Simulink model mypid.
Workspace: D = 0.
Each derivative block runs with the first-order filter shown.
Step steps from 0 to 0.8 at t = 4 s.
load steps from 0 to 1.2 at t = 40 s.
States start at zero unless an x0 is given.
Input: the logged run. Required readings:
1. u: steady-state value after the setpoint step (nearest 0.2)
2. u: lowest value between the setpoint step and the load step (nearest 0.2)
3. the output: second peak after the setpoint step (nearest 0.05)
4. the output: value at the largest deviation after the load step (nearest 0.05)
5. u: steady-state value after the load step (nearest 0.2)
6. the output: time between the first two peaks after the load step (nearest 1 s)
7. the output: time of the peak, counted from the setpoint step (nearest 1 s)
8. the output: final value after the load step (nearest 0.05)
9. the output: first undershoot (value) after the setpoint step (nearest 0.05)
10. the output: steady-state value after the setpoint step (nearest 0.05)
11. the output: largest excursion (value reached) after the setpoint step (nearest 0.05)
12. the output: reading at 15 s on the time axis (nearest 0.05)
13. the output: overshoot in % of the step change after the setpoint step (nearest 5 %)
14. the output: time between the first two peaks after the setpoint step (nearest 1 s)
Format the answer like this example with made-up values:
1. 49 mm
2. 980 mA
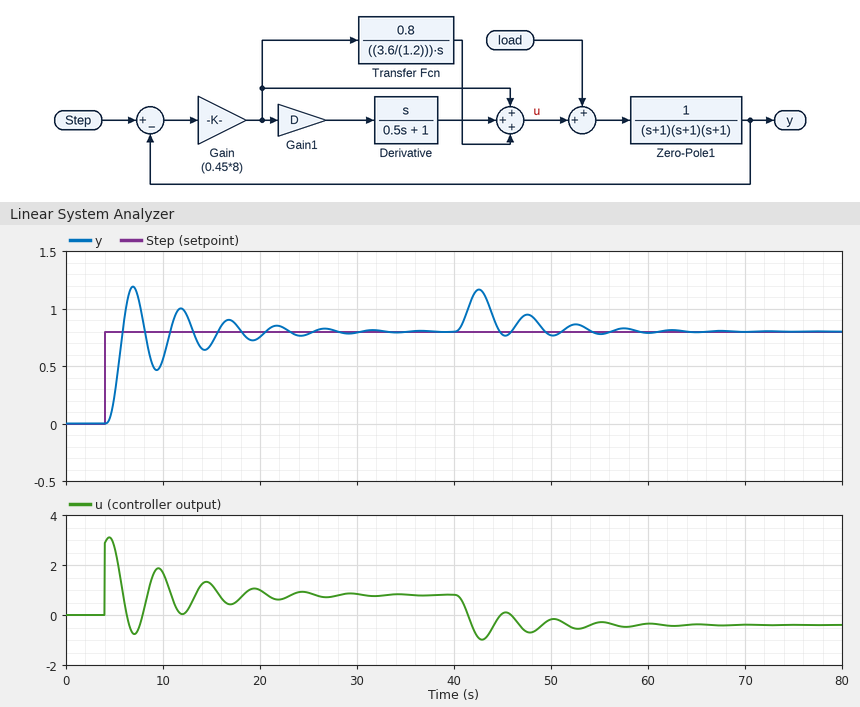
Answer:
1. 0.8
2. -0.8
3. 1.00
4. 1.15
5. -0.4
6. 5 s
7. 3 s
8. 0.80
9. 0.45
10. 0.80
11. 1.20
12. 0.70
13. 50 %
14. 5 s
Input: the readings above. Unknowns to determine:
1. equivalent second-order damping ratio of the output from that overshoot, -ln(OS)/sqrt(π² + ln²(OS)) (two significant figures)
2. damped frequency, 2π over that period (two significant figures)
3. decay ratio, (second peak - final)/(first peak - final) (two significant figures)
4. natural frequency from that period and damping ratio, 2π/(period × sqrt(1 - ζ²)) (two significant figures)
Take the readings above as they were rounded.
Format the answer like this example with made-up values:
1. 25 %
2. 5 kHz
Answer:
1. 0.22
2. 1.3 rad/s
3. 0.50
4. 1.3 rad/s
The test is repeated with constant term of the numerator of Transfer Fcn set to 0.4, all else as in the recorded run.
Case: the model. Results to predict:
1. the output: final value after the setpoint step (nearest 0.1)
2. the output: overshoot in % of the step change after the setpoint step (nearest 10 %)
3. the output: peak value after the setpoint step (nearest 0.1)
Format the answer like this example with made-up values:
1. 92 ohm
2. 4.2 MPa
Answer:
1. 0.8
2. 30 %
3. 1.1
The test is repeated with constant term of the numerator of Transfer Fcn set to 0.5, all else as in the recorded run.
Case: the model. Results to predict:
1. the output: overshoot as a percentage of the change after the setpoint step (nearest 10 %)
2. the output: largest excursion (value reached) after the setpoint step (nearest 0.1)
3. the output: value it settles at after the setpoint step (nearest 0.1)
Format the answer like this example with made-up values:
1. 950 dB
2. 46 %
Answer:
1. 40 %
2. 1.1
3. 0.8
